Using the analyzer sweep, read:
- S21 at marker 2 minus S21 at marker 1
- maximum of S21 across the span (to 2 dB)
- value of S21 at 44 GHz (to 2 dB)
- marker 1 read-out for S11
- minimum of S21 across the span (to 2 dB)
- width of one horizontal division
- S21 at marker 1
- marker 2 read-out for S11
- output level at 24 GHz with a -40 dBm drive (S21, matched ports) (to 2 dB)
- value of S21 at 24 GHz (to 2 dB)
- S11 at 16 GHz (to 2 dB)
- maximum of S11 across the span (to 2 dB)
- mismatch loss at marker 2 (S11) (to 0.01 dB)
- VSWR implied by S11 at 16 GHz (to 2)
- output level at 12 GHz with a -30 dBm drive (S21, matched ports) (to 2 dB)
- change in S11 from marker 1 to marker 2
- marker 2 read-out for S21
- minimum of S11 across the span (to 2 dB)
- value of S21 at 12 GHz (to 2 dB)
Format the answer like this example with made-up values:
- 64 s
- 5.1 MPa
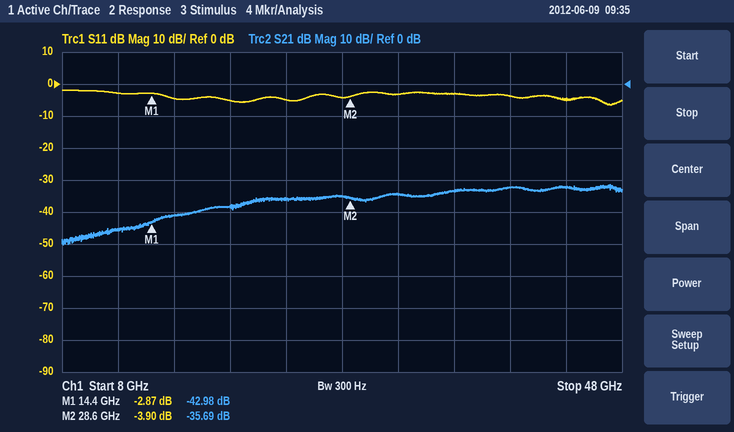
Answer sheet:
- 7.29 dB
- -32 dB
- -32 dB
- -2.87 dB
- -50 dB
- 4 GHz
- -42.98 dB
- -3.90 dB
- -76 dBm
- -36 dB
- -4 dB
- -2 dB
- 2.27 dB
- 4
- -76 dBm
- -1.03 dB
- -35.69 dB
- -6 dB
- -46 dB
